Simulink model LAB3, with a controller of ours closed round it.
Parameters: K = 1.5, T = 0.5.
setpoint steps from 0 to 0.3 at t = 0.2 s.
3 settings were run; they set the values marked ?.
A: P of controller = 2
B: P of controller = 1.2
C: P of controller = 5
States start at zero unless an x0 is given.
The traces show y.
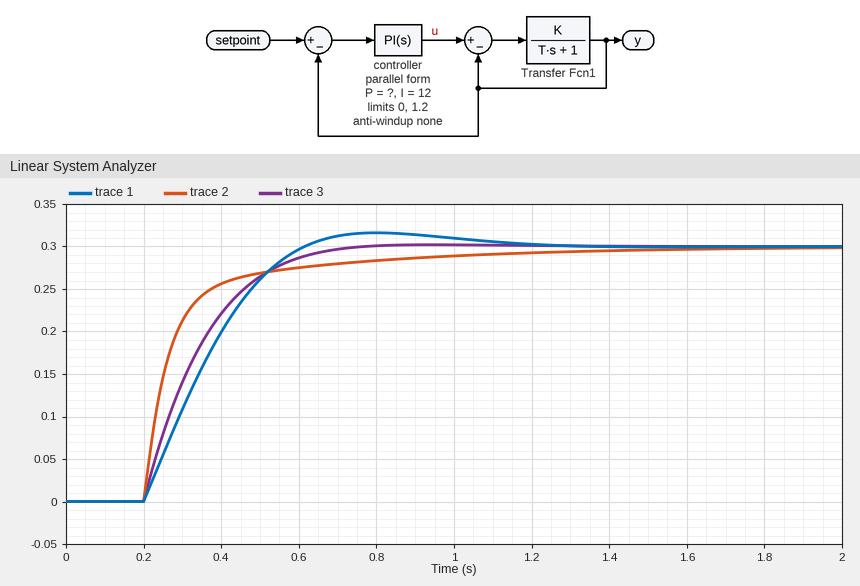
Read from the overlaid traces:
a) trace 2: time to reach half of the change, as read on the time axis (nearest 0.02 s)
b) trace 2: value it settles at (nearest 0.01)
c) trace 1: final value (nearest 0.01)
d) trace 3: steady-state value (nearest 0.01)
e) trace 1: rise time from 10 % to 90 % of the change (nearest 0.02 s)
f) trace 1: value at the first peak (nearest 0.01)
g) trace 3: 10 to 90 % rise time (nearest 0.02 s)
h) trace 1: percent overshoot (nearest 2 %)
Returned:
0.26 s
0.30
0.30
0.30
0.30 s
0.32
0.30 s
6 %
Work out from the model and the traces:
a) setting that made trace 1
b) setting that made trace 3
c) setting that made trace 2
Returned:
B
A
C
